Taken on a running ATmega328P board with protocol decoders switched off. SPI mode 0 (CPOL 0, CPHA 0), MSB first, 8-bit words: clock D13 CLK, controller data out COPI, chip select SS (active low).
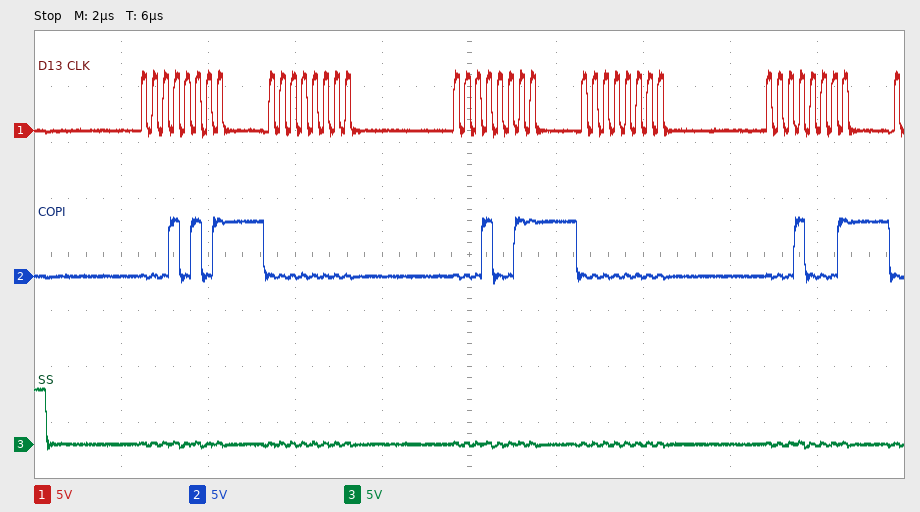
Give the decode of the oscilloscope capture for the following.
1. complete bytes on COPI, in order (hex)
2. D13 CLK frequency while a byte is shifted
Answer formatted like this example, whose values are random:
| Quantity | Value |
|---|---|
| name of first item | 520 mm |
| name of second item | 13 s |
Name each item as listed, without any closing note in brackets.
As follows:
| Quantity | Value |
|---|---|
| complete bytes on COPI, in order | 15 00 13 00 11 |
| D13 CLK frequency while a byte is shifted | 4 MHz |
